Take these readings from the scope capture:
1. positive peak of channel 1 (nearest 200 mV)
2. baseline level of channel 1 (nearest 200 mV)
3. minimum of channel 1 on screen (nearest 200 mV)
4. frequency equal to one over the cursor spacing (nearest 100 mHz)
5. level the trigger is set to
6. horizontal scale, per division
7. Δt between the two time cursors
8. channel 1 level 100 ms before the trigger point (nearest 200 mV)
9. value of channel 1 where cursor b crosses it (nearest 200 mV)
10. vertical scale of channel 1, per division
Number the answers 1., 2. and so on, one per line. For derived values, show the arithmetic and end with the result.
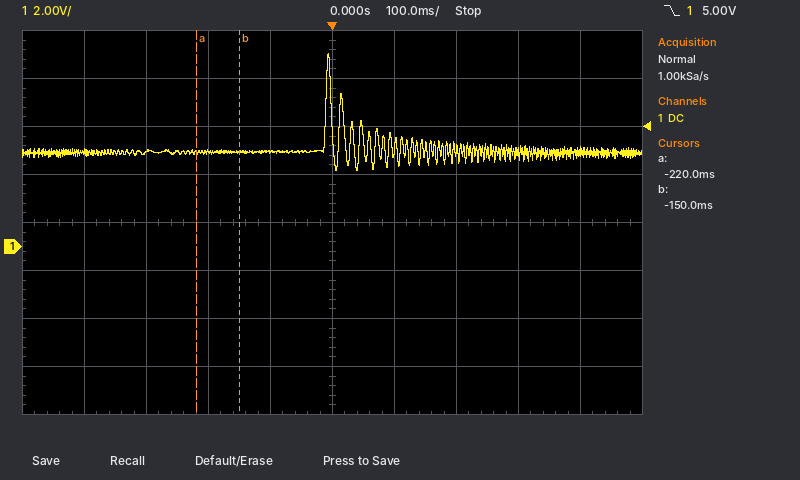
1. 8.0 V
2. 4.0 V
3. 3.2 V
4. 1 / 70 ms ≈ 14.3 Hz
5. 5.00 V
6. 100 ms
7. -150 ms − (-220 ms) = 70 ms
8. 4.0 V
9. 4.0 V
10. 2 V
